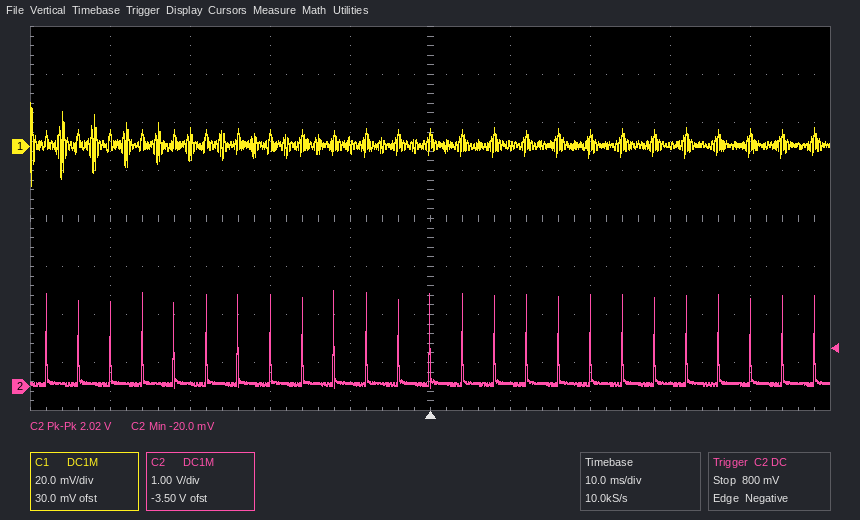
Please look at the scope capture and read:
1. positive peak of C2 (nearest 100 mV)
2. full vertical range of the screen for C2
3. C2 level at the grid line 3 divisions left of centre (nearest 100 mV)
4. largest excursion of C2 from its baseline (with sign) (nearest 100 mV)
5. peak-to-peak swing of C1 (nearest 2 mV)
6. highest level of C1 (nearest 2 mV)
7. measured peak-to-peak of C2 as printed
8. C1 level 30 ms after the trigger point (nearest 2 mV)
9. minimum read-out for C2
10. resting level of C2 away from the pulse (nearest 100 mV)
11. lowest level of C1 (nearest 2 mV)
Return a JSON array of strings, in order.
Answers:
["2.0 V", "8 V", "100 mV", "+1.9 V", "34 mV", "18 mV", "2.02 V", "0 mV", "-20.0 mV", "100 mV", "-16 mV"]
